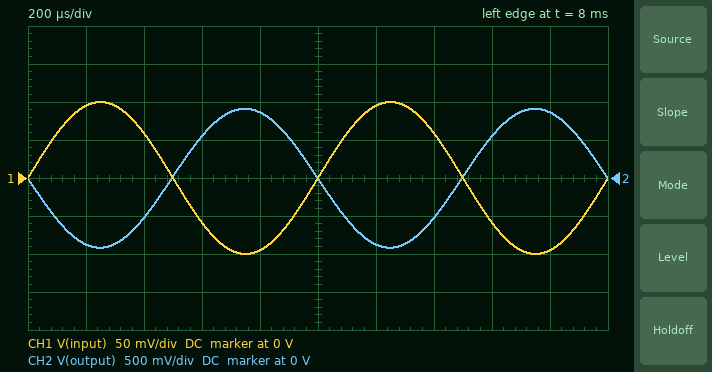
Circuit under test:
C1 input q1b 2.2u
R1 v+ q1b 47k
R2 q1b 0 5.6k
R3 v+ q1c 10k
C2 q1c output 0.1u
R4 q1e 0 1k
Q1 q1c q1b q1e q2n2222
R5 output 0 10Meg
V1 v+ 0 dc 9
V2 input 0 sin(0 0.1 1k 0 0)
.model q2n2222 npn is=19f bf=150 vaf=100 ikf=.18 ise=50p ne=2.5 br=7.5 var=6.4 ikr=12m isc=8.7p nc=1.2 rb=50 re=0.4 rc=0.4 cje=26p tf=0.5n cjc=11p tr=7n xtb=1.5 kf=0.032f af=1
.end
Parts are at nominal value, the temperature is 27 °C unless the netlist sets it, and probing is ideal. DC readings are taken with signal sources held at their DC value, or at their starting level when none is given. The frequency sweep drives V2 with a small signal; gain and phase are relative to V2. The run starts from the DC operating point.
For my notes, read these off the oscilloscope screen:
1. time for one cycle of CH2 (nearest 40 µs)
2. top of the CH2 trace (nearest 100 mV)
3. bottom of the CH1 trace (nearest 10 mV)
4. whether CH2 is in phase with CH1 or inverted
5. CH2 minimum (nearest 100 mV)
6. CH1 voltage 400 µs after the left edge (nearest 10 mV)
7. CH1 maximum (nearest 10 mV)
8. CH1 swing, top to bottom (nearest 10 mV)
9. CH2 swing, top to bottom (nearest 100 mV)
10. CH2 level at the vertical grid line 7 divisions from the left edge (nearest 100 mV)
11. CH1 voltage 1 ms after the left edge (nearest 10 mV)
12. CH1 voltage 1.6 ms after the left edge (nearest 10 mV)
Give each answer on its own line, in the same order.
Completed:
1.00 ms
900 mV
-100 mV
inverted
-900 mV
60 mV
100 mV
200 mV
1.8 V
-500 mV
0 V
-60 mV
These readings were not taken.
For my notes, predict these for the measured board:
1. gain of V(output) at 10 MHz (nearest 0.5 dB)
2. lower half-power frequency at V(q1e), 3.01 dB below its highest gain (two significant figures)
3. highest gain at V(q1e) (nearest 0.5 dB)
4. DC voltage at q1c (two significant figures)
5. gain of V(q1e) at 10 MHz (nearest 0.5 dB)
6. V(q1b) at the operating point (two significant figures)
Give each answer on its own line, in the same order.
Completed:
8.5 dB
16 Hz
-0.5 dB
5.7 V
-1.0 dB
940 mV
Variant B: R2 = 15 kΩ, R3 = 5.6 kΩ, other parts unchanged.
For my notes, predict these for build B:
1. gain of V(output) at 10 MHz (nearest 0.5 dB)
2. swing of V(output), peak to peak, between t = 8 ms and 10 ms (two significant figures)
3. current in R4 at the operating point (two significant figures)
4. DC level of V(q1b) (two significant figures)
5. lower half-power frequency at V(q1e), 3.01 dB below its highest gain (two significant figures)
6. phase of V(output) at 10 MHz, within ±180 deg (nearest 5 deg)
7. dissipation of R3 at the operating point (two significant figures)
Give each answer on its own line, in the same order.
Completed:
2.0 dB
780 mV
1.3 mA
2.0 V
46 Hz
60 deg
9.8 mW
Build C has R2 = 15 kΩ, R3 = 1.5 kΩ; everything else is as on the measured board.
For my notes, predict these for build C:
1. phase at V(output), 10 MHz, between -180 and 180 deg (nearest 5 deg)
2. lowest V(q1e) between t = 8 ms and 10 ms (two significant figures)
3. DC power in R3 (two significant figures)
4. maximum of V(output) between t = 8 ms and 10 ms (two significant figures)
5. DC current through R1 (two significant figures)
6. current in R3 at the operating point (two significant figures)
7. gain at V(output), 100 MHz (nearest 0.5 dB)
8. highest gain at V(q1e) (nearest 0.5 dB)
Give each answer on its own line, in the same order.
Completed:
125 deg
1.3 V
2.9 mW
150 mV
150 µA
1.4 mA
0.5 dB
0 dB
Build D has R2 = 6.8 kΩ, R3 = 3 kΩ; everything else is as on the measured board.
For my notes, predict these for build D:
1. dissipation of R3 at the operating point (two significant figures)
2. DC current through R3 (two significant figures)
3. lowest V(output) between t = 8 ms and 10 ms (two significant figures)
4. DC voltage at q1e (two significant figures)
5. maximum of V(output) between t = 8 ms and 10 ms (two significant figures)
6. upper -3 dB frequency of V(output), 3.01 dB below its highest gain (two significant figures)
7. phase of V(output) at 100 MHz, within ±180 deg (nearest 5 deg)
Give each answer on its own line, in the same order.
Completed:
710 µW
490 µA
-280 mV
490 mV
280 mV
12 MHz
10 deg
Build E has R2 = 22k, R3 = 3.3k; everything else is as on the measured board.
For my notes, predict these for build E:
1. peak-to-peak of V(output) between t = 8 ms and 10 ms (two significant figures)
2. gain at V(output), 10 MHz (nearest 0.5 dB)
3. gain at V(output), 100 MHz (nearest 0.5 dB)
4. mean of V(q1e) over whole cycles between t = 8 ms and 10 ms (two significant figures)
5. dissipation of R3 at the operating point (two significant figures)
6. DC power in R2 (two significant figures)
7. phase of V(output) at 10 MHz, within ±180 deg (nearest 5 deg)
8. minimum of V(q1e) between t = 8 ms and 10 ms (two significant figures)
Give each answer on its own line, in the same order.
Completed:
610 mV
3.5 dB
0 dB
2.0 V
13 mW
310 µW
75 deg
1.9 V
